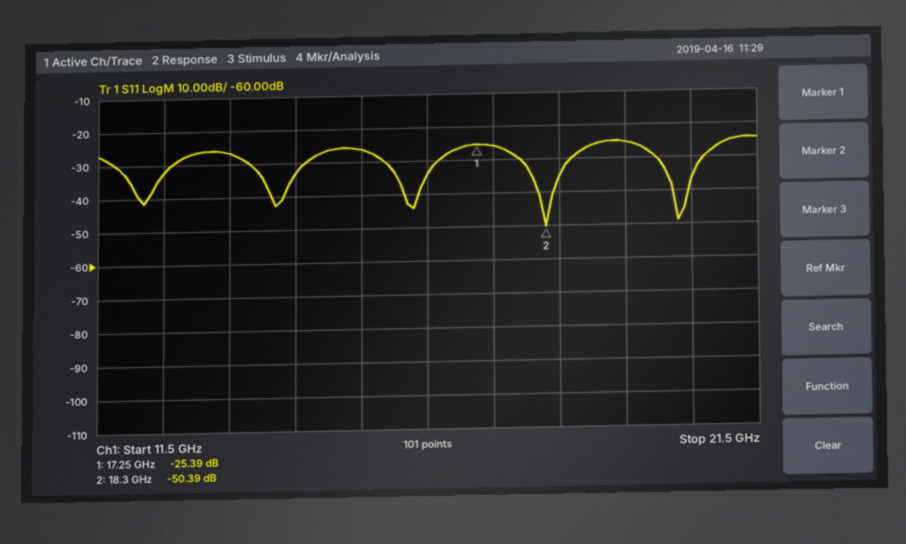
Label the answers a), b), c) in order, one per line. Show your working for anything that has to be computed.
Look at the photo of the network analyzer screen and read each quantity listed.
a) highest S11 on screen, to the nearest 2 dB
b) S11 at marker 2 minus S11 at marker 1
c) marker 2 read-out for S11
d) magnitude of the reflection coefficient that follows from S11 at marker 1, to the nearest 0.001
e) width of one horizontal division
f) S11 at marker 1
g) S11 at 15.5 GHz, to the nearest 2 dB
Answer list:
a) -24 dB
b) -50.39 − (-25.39) = -25.00 dB
c) -50.39 dB
d) 10^(-25.39/20) ≈ 0.054
e) 1 GHz
f) -25.39 dB
g) -26 dB
